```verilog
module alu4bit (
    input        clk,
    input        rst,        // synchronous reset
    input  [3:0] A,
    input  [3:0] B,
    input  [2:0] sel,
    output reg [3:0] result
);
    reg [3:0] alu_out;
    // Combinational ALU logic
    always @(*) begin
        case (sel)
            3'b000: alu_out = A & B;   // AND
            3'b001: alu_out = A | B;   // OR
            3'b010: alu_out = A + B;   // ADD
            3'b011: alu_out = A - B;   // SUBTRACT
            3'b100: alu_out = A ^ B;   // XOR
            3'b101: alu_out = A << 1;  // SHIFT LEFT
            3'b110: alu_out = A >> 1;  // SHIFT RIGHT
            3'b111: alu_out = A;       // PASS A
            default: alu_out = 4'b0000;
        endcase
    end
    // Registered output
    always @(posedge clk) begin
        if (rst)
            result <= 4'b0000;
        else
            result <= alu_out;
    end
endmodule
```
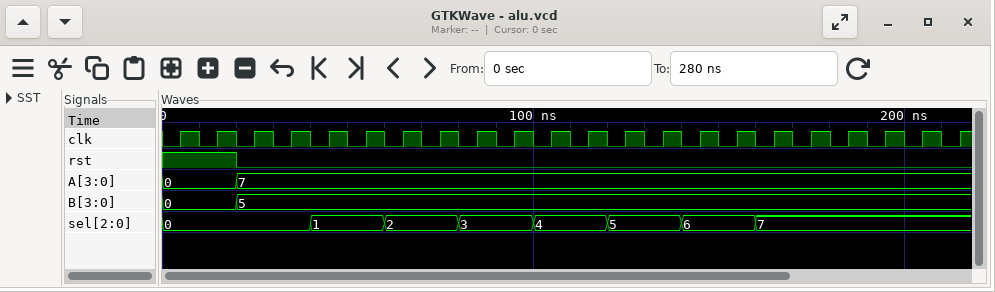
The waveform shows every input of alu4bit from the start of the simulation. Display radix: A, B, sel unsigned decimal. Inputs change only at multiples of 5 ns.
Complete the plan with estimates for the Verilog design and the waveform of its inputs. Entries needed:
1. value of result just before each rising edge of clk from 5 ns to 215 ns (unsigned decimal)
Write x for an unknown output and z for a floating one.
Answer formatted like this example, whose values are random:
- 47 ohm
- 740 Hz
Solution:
- x, 0, 0, 5, 5, 7, 7, 12, 12, 2, 2, 2, 2, 14, 14, 3, 3, 7, 7, 7, 7, 7
